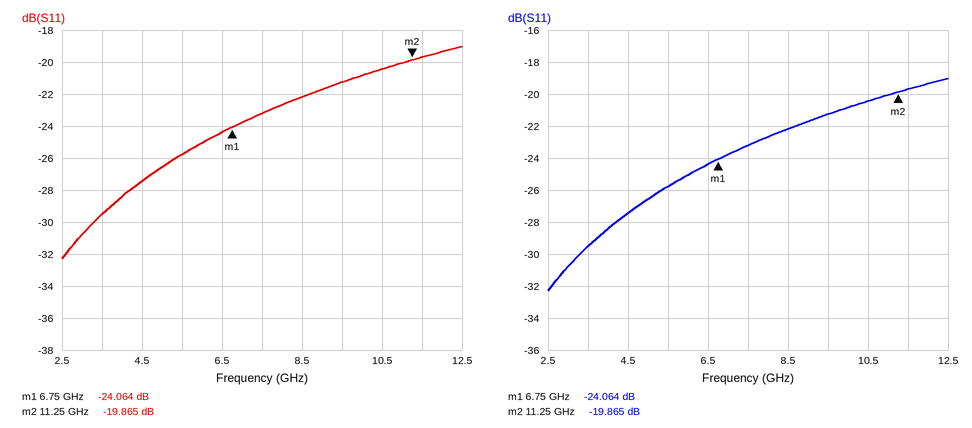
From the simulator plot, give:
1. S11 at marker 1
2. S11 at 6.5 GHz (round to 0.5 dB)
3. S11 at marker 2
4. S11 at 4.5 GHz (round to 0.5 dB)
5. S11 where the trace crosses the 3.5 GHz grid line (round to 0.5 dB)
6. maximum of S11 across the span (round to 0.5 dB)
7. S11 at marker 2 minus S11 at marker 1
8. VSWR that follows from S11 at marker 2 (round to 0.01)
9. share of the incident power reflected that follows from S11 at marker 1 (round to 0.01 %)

-24.064 dB
-24.5 dB
-19.865 dB
-27.5 dB
-29.5 dB
-19.0 dB
4.199 dB
1.23
0.39 %
